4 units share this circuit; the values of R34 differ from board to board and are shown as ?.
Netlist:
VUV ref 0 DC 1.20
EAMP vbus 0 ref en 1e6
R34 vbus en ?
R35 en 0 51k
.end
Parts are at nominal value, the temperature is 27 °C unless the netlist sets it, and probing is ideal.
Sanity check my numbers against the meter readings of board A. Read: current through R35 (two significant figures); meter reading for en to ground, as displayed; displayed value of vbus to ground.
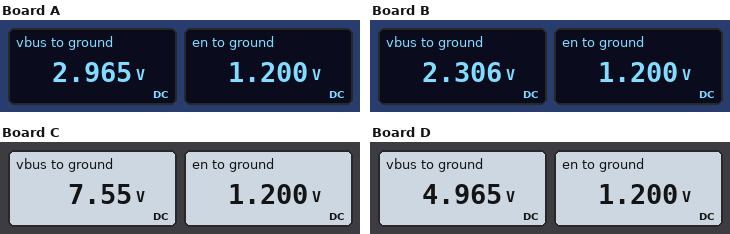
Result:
24 µA
1.200 V
2.965 V
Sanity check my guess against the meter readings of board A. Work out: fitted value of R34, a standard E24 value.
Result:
75 kΩ
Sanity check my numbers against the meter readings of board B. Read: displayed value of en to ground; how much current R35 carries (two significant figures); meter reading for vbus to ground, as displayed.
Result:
1.200 V
24 µA
2.306 V
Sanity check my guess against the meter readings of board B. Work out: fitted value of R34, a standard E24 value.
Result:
47 kΩ
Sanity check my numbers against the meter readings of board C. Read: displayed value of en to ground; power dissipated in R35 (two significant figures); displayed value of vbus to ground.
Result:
1.200 V
28 µW
7.55 V
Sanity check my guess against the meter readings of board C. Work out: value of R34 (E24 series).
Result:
270 kΩ
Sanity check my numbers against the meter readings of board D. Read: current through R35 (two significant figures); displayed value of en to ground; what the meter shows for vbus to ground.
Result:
24 µA
1.200 V
4.965 V
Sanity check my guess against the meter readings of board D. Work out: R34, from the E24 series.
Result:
160 kΩ
